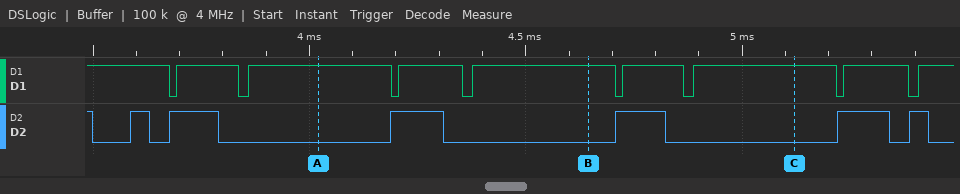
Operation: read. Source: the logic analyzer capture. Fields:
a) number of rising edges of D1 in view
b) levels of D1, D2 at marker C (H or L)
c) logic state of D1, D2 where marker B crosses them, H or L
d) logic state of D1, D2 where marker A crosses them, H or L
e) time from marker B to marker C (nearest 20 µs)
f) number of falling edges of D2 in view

8
D1=H, D2=L
D1=H, D2=L
D1=H, D2=L
480 µs
7
